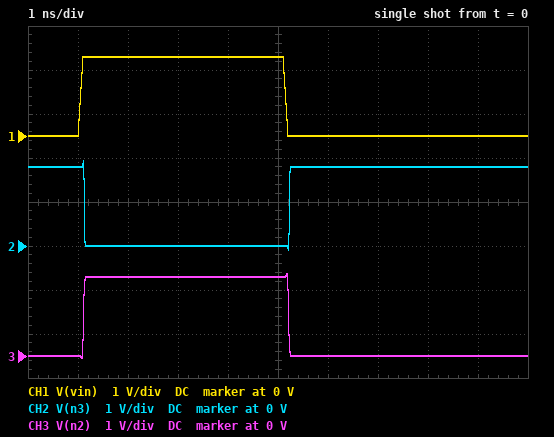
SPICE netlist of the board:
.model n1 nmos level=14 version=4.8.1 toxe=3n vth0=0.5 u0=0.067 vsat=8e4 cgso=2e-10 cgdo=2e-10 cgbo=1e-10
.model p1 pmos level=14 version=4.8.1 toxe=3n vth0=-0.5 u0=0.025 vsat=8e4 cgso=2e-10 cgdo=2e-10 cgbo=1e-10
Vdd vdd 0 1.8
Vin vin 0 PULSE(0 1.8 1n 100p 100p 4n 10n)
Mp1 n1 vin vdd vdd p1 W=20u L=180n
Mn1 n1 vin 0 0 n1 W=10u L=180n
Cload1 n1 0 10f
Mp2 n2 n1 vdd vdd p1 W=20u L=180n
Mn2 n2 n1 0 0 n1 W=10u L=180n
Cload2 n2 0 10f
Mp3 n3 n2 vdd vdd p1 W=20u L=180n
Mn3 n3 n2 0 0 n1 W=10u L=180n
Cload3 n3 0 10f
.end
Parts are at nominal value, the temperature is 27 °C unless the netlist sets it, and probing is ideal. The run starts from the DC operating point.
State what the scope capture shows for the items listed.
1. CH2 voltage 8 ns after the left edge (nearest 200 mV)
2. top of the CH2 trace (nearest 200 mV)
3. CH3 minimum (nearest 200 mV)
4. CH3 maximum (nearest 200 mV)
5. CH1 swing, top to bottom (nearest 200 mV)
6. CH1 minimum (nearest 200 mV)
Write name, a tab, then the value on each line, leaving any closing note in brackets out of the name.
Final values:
CH2 voltage 8 ns after the left edge	1.8 V
top of the CH2 trace	2.0 V
CH3 minimum	0 V
CH3 maximum	1.8 V
CH1 swing, top to bottom	1.8 V
CH1 minimum	0 V
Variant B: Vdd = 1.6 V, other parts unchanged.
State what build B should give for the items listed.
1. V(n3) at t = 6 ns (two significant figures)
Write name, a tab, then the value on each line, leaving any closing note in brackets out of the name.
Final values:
V(n3) at t = 6 ns	1.6 V
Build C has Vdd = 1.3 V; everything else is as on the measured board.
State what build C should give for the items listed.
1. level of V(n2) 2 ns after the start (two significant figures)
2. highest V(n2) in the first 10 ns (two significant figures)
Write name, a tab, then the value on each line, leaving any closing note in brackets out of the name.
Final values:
level of V(n2) 2 ns after the start	1.3 V
highest V(n2) in the first 10 ns	1.4 V
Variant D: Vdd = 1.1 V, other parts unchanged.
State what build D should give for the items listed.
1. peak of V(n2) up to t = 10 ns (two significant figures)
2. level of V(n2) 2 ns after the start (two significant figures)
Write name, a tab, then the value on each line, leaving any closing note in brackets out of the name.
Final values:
peak of V(n2) up to t = 10 ns	1.2 V
level of V(n2) 2 ns after the start	1.1 V
